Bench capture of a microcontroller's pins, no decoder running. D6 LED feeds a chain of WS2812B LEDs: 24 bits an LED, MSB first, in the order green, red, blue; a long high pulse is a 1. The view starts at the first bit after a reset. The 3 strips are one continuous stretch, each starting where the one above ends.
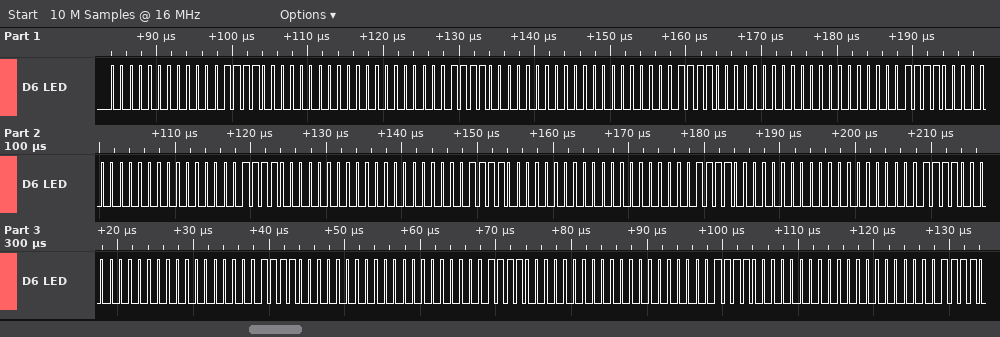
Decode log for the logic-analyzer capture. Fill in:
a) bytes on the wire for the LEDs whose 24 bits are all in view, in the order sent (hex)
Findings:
00 0F 00 00 0F 00 00 0F 00 00 0F 00 00 0F 00 00 0F 00 00 0F 00 00 0F 00 00 0F 00 00 0F 00 00 0F 00
